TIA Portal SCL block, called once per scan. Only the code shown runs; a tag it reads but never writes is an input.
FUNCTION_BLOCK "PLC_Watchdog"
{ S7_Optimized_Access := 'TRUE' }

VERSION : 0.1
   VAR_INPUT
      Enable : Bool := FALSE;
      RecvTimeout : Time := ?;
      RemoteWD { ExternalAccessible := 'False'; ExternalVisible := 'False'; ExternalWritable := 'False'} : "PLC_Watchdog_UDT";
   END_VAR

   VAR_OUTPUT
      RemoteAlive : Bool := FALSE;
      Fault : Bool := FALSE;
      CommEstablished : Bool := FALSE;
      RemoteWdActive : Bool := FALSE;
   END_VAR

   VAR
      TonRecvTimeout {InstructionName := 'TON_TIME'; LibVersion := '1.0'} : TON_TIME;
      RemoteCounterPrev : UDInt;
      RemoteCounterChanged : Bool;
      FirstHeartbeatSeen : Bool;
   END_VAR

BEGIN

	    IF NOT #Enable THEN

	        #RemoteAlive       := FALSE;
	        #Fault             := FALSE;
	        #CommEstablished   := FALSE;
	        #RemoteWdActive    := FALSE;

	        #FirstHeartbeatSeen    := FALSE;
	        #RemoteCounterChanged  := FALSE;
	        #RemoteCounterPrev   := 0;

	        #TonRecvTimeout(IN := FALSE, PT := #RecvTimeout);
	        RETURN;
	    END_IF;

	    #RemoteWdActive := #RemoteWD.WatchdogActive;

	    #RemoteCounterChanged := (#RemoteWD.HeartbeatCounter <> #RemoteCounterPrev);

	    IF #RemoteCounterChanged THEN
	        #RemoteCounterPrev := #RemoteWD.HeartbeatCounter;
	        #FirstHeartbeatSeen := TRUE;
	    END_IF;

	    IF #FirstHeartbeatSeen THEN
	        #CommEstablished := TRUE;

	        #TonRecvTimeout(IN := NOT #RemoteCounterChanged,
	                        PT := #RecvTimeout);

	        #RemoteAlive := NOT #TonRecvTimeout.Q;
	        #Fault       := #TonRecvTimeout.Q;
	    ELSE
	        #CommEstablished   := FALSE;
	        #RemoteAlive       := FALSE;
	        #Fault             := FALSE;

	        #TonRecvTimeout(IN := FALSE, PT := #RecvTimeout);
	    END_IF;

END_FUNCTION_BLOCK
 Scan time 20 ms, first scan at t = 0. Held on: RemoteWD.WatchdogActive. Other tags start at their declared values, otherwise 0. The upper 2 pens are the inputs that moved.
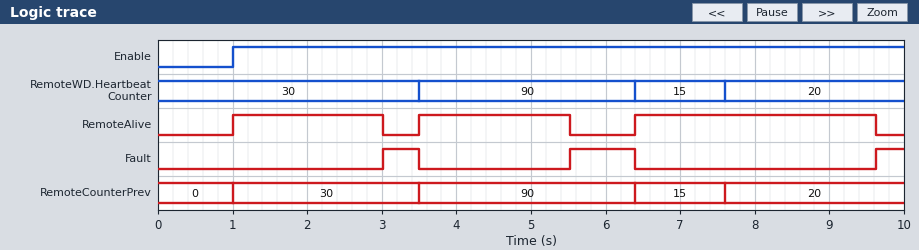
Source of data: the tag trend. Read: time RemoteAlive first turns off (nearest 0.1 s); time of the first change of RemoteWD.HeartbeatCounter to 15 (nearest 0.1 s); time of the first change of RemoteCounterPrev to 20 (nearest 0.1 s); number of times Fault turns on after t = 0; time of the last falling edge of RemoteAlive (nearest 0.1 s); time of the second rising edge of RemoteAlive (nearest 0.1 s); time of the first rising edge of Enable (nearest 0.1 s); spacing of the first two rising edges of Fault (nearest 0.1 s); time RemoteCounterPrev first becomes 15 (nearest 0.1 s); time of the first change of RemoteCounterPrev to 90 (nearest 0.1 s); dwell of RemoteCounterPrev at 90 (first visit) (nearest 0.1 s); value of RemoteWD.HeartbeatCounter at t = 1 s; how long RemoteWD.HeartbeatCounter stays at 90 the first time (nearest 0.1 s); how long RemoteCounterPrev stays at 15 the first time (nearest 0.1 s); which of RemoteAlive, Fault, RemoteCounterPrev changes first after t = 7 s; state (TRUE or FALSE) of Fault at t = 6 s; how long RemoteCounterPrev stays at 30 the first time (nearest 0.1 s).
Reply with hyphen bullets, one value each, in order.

- 3.0 s
- 6.4 s
- 7.6 s
- 3
- 9.6 s
- 3.5 s
- 1.0 s
- 2.5 s
- 6.4 s
- 3.5 s
- 2.9 s
- 30
- 2.9 s
- 1.2 s
- RemoteCounterPrev
- TRUE
- 2.5 s
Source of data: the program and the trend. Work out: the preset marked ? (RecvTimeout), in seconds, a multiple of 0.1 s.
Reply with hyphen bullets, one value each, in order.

- 2.0 s
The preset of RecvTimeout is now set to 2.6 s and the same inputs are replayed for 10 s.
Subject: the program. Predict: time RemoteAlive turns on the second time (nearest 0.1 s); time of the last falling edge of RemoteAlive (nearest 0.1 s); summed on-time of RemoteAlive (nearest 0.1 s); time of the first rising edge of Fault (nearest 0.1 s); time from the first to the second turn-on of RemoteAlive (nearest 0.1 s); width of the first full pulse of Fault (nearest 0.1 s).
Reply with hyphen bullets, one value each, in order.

- 6.4 s
- 6.1 s
- 8.7 s
- 6.1 s
- 5.4 s
- 0.3 s
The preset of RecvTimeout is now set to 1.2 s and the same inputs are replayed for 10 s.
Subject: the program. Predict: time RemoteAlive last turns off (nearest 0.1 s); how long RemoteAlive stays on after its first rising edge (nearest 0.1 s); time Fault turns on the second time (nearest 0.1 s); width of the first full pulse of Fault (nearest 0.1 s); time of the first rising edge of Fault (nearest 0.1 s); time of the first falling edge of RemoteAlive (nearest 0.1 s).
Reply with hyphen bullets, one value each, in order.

- 8.8 s
- 1.2 s
- 4.7 s
- 1.3 s
- 2.2 s
- 2.2 s
